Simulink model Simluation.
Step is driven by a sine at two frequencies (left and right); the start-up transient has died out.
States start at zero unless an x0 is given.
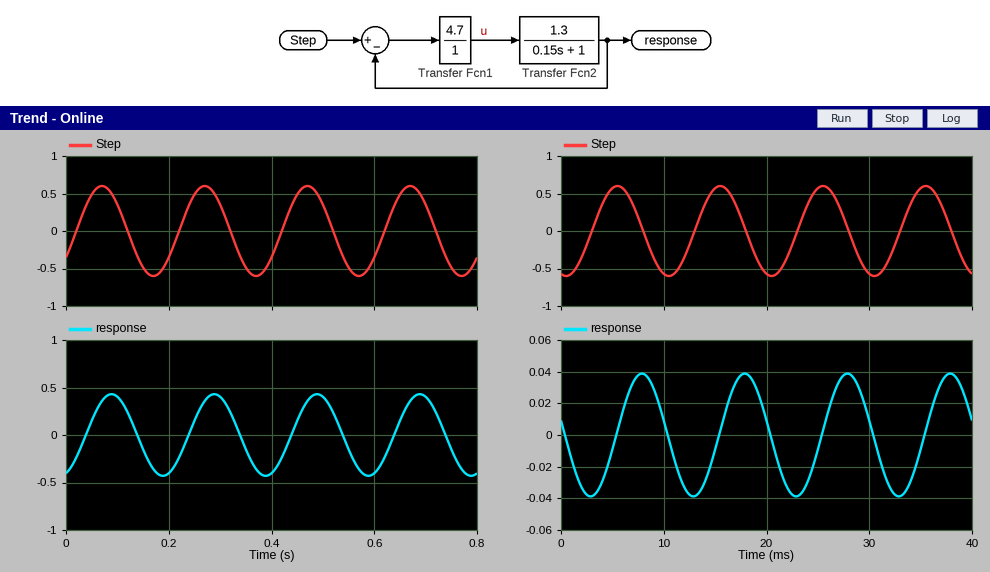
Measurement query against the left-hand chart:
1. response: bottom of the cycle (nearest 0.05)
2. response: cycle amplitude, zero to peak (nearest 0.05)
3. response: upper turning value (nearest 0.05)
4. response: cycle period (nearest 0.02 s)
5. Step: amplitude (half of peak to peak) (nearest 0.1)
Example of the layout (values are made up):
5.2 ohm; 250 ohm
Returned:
-0.45; 0.45; 0.45; 0.20 s; 0.6
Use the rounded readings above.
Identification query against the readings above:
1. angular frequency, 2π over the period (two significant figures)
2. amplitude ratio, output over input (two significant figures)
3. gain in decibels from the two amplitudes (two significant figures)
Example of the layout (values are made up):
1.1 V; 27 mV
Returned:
31 rad/s; 0.75; -2.5 dB
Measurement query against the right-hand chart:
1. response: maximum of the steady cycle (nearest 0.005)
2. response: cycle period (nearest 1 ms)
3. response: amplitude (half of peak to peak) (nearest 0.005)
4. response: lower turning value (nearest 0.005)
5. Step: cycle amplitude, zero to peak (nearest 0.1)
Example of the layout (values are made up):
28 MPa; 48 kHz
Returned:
0.040; 10 ms; 0.040; -0.040; 0.6
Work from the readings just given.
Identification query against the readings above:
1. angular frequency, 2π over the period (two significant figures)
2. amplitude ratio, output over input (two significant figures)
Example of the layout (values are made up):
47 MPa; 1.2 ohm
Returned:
0.63 rad/ms; 0.067
